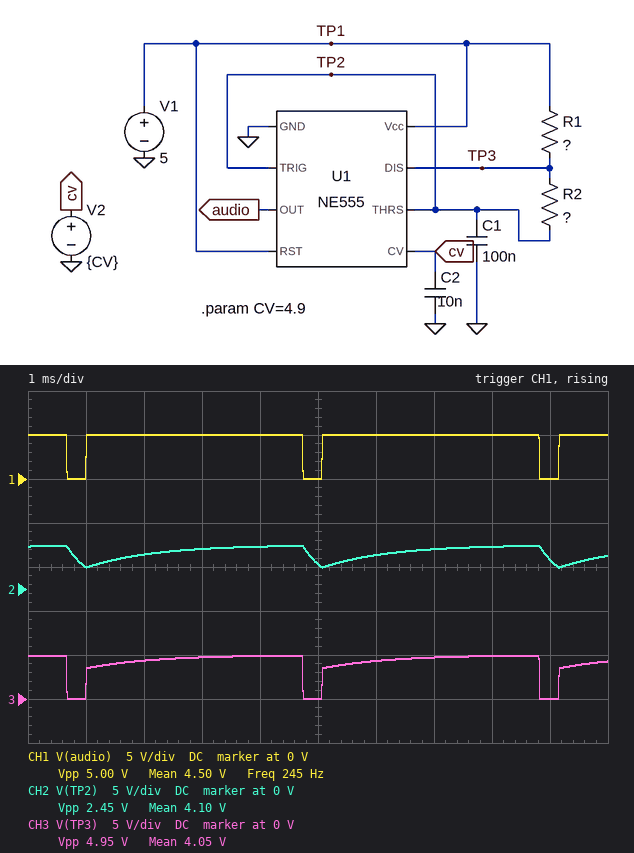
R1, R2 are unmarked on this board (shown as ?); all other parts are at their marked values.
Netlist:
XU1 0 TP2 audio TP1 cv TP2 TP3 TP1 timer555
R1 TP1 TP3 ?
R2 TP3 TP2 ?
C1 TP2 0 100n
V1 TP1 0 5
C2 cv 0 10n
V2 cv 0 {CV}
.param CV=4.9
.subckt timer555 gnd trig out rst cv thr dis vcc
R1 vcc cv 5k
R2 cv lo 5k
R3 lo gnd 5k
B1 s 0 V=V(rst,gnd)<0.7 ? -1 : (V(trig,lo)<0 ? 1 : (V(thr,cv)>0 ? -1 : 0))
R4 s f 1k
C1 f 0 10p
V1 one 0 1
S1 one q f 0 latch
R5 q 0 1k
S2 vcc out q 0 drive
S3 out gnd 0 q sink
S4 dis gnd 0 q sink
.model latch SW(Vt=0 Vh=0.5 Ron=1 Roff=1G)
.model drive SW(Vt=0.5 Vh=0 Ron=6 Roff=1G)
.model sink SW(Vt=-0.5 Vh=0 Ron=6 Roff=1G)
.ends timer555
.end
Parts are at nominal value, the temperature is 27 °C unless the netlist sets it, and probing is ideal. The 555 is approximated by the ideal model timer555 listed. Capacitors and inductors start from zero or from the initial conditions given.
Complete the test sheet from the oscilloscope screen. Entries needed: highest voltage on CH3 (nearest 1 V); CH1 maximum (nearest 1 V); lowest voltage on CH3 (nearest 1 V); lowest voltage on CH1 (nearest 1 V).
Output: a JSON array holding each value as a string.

["5 V", "5 V", "0 V", "0 V"]
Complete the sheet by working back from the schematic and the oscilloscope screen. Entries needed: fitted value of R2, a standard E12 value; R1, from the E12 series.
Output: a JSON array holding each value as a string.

["4.7 kΩ", "6.8 kΩ"]
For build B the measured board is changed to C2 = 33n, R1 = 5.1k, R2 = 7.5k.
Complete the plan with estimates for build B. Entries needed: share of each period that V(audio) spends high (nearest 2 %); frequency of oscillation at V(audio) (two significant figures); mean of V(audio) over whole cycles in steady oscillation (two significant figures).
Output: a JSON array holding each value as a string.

["88 %", "220 Hz", "4.4 V"]
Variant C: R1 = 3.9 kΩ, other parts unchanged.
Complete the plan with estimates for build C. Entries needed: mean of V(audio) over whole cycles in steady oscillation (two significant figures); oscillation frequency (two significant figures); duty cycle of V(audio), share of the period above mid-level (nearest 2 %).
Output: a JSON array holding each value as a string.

["4.5 V", "320 Hz", "90 %"]
